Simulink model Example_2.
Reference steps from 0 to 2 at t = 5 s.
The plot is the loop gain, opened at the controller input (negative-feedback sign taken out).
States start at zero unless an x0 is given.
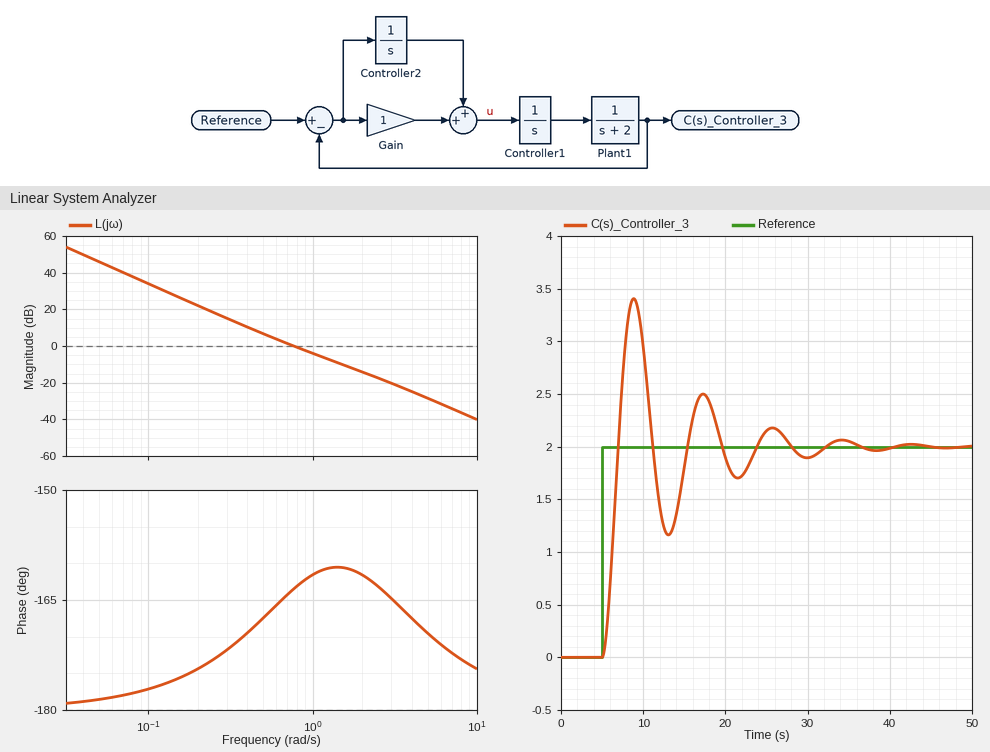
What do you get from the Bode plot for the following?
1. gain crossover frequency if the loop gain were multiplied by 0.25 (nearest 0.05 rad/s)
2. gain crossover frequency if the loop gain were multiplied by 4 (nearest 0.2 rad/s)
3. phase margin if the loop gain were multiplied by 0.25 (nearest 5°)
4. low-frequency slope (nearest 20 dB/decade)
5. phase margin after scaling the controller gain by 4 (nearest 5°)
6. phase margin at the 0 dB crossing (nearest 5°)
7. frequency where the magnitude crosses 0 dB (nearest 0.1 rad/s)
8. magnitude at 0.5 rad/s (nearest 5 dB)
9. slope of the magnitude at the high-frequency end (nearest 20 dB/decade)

0.35 rad/s
1.8 rad/s
10°
-40 dB/decade
20°
15°
0.8 rad/s
5 dB
-40 dB/decade
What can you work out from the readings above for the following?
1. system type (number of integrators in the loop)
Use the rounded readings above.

2
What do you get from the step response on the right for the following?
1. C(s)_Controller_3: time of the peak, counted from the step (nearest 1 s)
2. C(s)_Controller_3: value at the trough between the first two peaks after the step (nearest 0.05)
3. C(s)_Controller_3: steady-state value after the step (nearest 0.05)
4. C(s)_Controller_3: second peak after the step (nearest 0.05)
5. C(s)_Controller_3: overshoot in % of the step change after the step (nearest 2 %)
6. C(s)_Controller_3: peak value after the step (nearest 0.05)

4 s
1.15
2.00
2.50
70 %
3.40
